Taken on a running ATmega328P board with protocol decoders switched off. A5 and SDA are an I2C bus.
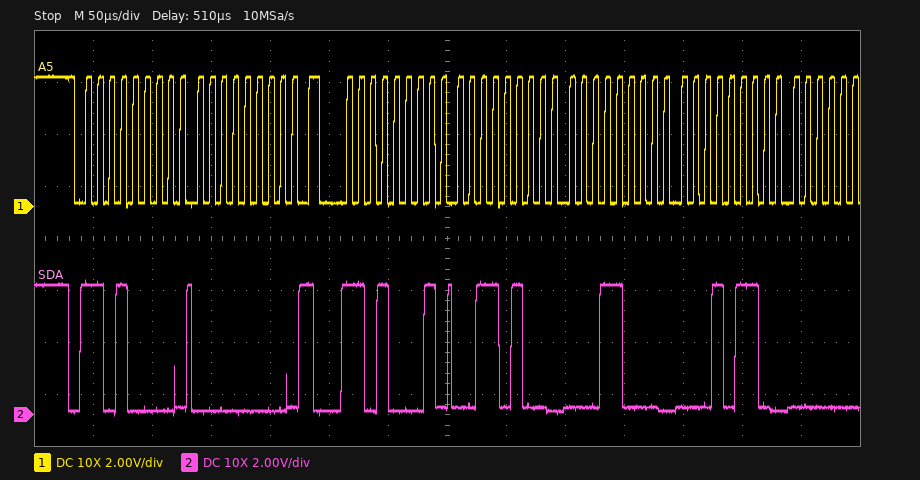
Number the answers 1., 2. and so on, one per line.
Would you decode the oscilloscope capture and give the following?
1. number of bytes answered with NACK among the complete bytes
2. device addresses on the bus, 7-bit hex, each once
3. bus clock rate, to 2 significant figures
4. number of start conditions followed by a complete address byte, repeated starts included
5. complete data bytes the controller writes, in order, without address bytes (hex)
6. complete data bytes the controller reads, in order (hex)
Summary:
1. 0
2. 0x68
3. 100 kHz
4. 2
5. 00
6. 34 18 16
